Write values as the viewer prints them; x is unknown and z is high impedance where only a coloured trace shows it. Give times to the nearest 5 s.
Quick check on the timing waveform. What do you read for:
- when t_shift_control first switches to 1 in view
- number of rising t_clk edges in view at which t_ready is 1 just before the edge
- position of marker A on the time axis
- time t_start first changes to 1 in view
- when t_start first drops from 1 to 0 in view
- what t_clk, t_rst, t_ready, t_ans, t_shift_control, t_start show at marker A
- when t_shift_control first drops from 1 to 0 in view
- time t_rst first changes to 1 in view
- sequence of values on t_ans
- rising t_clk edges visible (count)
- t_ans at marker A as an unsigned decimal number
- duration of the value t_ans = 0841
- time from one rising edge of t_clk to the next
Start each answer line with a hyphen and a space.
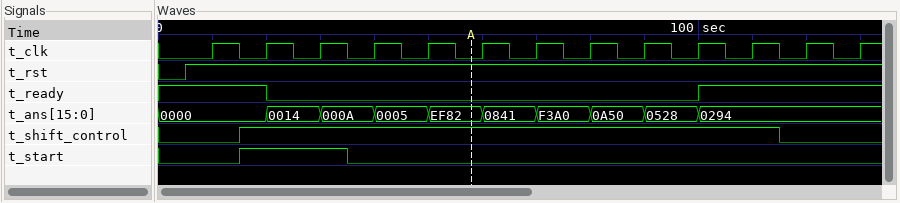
- 15 s
- 5
- 60 s
- 15 s
- 35 s
- t_clk=0, t_rst=1, t_ready=0, t_ans=EF82, t_shift_control=1, t_start=0
- 115 s
- 5 s
- 0000, 0014, 000A, 0005, EF82, 0841, F3A0, 0A50, 0528, 0294
- 13
- 61314
- 10 s
- 10 s
